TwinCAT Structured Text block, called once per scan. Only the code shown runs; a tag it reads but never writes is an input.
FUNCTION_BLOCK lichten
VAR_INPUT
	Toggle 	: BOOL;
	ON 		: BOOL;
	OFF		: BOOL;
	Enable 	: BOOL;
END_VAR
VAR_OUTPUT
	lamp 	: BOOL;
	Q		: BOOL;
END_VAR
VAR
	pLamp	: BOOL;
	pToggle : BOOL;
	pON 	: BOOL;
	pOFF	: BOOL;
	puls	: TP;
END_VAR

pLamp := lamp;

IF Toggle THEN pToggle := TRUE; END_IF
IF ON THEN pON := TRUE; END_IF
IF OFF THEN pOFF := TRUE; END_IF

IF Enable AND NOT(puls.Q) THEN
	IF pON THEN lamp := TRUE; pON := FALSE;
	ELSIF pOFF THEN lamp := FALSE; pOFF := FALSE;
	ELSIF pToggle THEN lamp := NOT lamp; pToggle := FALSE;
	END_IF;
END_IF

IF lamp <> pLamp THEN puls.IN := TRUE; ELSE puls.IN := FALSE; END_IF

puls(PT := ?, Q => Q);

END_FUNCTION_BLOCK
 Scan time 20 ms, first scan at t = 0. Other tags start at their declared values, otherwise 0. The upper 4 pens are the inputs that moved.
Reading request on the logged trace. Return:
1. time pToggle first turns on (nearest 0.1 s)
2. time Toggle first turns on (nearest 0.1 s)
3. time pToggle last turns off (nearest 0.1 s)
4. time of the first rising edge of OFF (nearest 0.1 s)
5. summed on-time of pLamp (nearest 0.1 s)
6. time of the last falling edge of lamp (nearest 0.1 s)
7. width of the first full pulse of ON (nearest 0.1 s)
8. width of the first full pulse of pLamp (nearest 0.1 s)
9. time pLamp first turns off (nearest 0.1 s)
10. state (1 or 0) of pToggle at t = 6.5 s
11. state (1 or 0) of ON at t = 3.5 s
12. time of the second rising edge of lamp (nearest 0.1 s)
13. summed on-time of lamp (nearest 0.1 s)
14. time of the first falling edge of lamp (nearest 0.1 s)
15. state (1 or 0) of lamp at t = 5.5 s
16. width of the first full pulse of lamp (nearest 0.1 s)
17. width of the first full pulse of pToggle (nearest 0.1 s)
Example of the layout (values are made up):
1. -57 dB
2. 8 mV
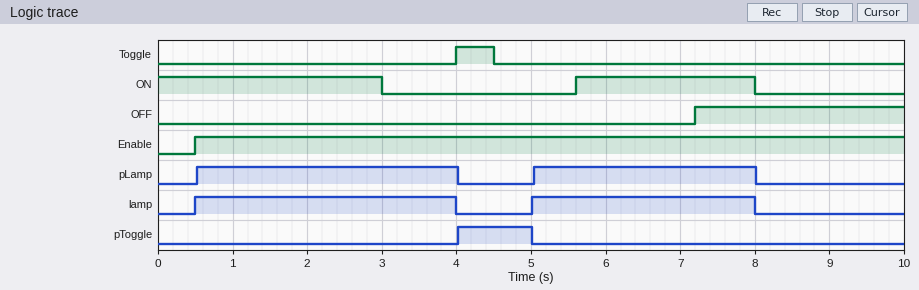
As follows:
1. 4.0 s
2. 4.0 s
3. 5.0 s
4. 7.2 s
5. 6.5 s
6. 8.0 s
7. 2.4 s
8. 3.5 s
9. 4.0 s
10. 0
11. 0
12. 5.0 s
13. 6.5 s
14. 4.0 s
15. 1
16. 3.5 s
17. 1.0 s
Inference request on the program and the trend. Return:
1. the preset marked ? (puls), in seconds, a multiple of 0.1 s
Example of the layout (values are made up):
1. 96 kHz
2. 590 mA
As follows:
1. 1.0 s
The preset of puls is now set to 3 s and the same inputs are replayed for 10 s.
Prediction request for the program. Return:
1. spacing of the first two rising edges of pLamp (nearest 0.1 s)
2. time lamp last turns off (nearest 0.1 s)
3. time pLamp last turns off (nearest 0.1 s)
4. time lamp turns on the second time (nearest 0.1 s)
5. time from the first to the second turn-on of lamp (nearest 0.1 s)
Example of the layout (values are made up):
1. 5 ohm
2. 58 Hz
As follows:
1. 6.5 s
2. 4.0 s
3. 4.0 s
4. 7.0 s
5. 6.5 s
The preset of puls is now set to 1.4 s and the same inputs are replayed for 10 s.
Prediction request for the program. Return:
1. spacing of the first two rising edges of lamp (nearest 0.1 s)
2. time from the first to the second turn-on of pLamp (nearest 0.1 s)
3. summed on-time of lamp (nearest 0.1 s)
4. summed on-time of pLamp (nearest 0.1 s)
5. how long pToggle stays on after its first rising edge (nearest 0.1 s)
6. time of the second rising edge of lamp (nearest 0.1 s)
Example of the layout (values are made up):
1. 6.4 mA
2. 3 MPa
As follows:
1. 4.9 s
2. 4.9 s
3. 6.1 s
4. 6.1 s
5. 1.4 s
6. 5.4 s
